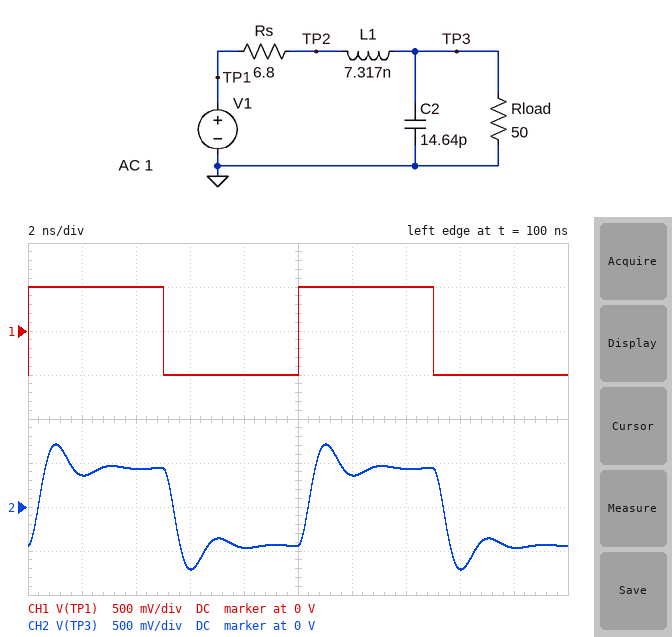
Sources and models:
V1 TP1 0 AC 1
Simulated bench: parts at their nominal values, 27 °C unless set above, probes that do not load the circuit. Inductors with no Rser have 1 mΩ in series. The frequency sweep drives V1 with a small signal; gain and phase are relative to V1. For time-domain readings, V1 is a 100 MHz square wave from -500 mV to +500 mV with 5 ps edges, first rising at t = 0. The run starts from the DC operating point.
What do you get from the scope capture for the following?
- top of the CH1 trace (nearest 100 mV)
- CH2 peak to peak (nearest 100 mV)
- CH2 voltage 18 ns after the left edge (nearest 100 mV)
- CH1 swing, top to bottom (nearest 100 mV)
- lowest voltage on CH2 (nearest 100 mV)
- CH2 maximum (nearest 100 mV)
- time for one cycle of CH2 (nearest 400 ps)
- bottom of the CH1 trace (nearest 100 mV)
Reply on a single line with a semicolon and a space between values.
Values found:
500 mV; 1.4 V; -500 mV; 1.0 V; -700 mV; 700 mV; 10.0 ns; -500 mV
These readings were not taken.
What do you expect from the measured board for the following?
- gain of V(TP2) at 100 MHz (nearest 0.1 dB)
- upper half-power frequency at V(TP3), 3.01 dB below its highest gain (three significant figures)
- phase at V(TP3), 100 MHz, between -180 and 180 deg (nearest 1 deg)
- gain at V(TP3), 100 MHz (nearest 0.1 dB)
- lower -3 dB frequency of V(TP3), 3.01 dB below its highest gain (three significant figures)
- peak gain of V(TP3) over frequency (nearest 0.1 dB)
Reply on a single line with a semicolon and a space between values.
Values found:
-1.2 dB; 616 MHz; -8 deg; -0.9 dB; 157 MHz; 2.5 dB
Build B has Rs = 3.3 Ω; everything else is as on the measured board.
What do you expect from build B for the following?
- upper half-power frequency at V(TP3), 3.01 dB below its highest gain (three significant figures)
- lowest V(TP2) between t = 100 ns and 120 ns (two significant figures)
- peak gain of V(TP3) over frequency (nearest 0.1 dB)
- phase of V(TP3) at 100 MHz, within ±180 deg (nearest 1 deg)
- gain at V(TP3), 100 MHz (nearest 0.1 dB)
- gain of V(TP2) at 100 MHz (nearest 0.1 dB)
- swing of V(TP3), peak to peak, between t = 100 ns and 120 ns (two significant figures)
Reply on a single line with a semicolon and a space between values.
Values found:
591 MHz; -530 mV; 4.6 dB; -7 deg; -0.3 dB; -0.6 dB; 1.7 V
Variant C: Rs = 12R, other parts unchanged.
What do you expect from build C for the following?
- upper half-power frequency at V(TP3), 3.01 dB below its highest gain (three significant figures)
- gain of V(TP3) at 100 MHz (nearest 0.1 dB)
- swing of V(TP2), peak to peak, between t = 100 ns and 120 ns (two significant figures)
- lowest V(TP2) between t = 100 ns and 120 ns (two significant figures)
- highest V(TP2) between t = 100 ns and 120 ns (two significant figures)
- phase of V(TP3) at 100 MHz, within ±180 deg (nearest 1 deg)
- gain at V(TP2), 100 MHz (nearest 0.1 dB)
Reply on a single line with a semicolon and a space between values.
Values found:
641 MHz; -1.7 dB; 1.2 V; -590 mV; 590 mV; -10 deg; -2.0 dB
